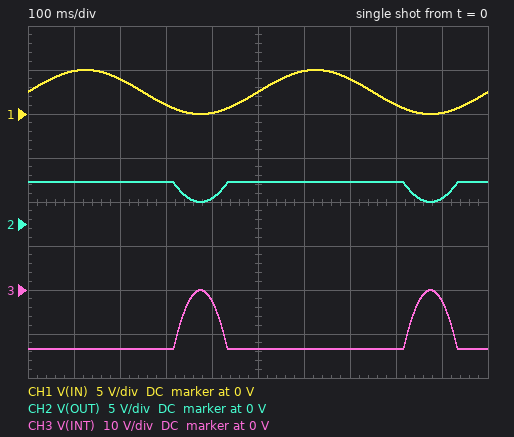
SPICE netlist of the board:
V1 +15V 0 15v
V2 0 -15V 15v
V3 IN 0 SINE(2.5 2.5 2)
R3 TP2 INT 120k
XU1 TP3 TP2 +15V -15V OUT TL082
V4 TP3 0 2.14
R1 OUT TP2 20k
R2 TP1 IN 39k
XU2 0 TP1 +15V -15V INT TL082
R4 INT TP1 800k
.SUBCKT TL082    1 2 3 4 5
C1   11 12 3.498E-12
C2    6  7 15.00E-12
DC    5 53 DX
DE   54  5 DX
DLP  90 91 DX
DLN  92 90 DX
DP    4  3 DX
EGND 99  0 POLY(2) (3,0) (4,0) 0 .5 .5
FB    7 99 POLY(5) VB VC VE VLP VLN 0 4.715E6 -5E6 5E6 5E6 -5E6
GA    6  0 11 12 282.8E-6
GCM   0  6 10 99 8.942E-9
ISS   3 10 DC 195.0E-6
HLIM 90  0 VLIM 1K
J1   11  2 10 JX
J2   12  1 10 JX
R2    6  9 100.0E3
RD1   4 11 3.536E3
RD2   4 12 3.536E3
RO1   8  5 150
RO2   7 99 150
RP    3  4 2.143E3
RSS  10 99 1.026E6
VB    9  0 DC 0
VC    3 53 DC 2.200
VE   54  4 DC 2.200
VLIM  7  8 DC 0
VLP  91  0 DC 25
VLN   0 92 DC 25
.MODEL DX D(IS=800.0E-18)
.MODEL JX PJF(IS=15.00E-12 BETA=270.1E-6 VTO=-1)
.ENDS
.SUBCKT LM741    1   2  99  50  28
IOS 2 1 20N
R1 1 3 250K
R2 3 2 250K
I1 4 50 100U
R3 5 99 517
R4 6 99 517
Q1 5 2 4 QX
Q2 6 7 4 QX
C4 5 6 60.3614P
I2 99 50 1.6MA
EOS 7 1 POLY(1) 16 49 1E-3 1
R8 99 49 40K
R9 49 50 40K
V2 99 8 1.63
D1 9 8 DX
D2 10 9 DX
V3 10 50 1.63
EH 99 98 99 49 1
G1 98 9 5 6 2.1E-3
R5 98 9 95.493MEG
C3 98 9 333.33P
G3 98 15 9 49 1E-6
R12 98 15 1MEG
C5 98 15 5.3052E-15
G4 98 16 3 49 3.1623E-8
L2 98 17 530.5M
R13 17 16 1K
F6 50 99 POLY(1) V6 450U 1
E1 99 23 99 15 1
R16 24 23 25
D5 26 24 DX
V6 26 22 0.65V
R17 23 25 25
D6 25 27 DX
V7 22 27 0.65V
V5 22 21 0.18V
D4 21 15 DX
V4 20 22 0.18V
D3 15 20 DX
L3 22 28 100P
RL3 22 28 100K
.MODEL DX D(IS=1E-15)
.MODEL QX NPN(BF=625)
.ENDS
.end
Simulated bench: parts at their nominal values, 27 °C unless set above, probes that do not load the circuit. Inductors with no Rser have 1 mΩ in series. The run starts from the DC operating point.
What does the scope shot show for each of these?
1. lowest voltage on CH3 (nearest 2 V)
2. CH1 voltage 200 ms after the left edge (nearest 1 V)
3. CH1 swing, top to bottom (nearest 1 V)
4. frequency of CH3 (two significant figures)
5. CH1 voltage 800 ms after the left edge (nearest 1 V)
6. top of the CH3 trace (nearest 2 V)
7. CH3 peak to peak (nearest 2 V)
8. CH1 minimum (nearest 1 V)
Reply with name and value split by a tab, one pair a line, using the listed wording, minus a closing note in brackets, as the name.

lowest voltage on CH3	-14 V
CH1 voltage 200 ms after the left edge	4 V
CH1 swing, top to bottom	5 V
frequency of CH3	2.0 Hz
CH1 voltage 800 ms after the left edge	1 V
top of the CH3 trace	0 V
CH3 peak to peak	14 V
CH1 minimum	0 V
